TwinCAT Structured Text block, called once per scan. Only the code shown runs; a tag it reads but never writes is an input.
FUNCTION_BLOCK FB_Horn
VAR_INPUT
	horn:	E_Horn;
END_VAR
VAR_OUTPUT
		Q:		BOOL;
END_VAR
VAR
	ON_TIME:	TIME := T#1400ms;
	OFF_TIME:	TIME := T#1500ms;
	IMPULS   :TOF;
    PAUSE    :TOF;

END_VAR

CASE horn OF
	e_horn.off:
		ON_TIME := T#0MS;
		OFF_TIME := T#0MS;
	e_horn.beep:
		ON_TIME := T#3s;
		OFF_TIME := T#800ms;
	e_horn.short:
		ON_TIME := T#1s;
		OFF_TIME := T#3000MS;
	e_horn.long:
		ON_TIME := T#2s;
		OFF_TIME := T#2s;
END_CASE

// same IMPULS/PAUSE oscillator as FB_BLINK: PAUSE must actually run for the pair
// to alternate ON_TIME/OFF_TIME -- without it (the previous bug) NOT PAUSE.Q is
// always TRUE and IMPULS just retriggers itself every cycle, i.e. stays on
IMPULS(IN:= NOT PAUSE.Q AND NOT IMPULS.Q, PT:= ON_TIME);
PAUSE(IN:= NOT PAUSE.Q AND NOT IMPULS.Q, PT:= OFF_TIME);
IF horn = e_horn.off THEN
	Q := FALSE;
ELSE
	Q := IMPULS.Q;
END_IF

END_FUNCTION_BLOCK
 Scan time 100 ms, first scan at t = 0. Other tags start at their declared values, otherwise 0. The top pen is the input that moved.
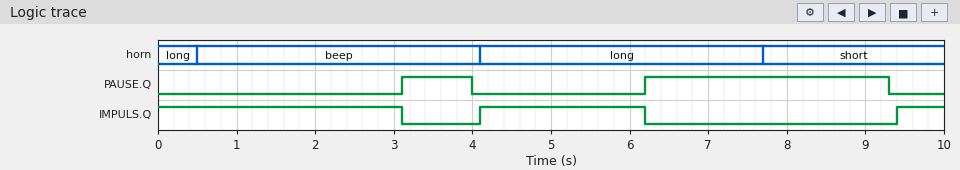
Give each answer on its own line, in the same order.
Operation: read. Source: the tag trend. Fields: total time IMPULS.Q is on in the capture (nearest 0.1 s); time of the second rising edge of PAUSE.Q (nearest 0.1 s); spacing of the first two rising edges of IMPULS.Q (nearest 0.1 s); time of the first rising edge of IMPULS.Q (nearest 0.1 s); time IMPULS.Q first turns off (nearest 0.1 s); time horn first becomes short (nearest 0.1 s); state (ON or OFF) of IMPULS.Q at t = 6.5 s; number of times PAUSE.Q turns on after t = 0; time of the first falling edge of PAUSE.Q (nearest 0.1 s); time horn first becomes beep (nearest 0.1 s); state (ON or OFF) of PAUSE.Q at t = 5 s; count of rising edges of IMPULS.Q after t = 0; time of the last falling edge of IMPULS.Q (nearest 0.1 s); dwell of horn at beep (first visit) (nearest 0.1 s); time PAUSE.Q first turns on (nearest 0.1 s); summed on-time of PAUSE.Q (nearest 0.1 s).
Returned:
5.8 s
6.2 s
5.3 s
4.1 s
3.1 s
7.7 s
OFF
2
4.0 s
0.5 s
OFF
2
6.2 s
3.6 s
3.1 s
4.0 s
